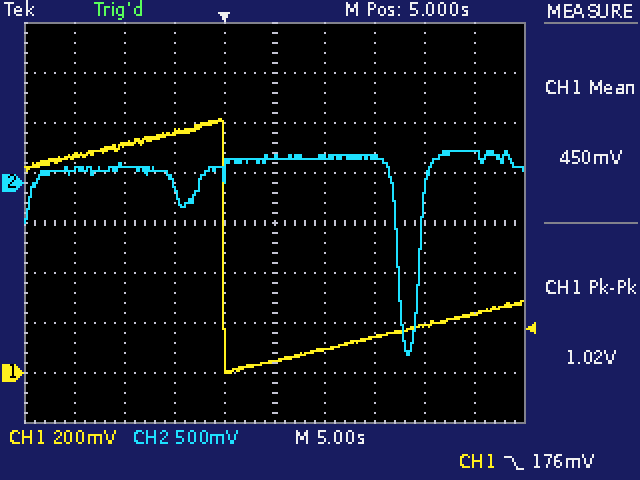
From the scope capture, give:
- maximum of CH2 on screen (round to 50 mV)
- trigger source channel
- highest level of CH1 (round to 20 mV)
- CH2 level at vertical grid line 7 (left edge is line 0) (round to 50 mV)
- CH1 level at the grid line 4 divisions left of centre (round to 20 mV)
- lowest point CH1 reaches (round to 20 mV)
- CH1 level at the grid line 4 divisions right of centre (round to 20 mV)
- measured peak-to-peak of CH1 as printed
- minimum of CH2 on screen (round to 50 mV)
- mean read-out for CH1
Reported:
300 mV
CH1
1.02 V
250 mV
860 mV
0 mV
240 mV
1.02 V
-1.70 V
450 mV
